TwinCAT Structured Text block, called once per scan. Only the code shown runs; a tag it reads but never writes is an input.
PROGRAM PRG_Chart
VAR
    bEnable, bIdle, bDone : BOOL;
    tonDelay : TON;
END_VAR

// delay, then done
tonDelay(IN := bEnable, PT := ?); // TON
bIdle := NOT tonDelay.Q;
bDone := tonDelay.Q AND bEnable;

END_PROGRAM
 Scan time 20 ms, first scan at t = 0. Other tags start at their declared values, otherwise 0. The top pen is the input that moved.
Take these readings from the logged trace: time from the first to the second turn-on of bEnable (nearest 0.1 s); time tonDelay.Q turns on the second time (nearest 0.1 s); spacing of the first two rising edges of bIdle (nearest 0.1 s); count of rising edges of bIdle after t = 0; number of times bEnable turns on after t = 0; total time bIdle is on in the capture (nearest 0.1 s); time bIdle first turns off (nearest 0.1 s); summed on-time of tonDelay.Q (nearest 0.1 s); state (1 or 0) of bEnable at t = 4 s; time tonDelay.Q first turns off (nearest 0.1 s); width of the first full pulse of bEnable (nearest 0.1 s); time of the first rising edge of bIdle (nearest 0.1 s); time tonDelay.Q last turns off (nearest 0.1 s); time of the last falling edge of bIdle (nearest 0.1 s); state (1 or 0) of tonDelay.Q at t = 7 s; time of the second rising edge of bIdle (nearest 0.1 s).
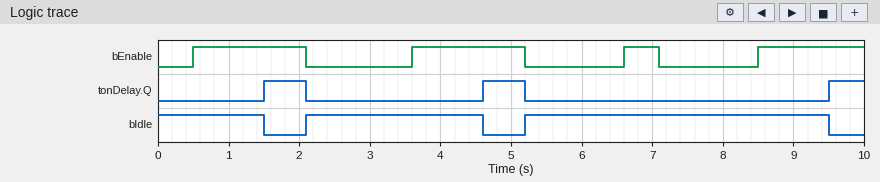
3.1 s
4.6 s
3.1 s
2
4
8.3 s
1.5 s
1.7 s
1
2.1 s
1.6 s
2.1 s
5.2 s
9.5 s
0
5.2 s
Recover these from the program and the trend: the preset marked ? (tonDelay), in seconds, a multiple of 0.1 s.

1.0 s
